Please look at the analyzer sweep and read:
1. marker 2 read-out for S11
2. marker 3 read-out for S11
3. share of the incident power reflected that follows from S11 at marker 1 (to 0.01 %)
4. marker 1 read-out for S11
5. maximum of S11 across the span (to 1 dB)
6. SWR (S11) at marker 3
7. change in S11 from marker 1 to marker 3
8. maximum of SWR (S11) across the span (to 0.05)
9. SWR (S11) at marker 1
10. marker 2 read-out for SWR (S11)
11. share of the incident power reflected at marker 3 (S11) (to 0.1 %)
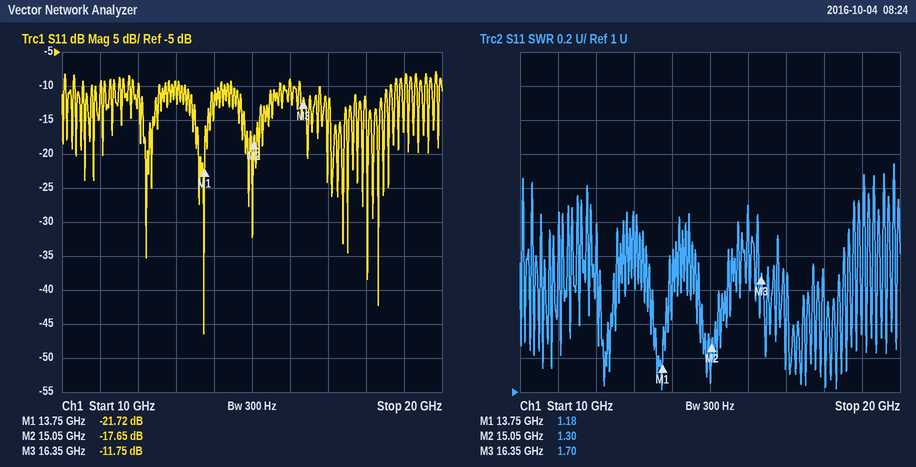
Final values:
-17.65 dB
-11.75 dB
0.67 %
-21.72 dB
-8 dB
1.70
9.97 dB
2.35
1.18
1.30
6.7 %
